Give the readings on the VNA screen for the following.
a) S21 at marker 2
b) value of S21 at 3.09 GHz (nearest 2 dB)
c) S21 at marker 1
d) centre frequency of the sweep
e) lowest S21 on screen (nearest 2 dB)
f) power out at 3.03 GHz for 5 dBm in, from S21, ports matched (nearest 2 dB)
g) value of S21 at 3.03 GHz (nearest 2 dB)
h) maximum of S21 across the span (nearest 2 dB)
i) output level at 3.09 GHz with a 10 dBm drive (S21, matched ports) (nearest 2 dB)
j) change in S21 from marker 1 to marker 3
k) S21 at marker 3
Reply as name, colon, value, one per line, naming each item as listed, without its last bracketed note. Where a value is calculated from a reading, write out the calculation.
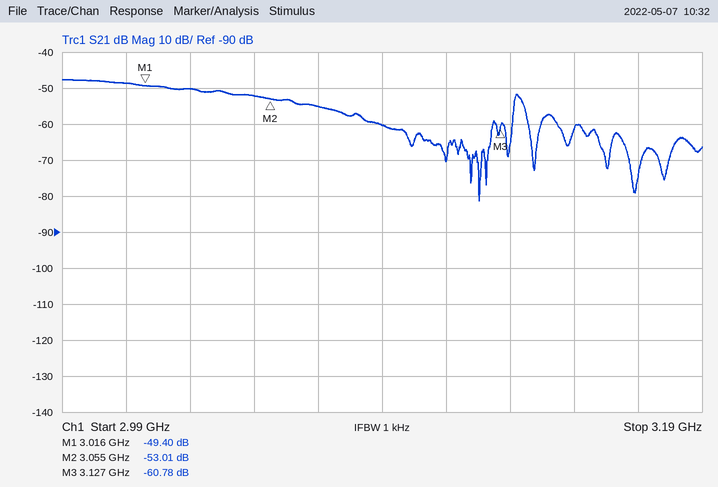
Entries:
S21 at marker 2: -53.01 dB
value of S21 at 3.09 GHz: -60 dB
S21 at marker 1: -49.40 dB
centre frequency of the sweep: 3.09 GHz
lowest S21 on screen: -82 dB
power out at 3.03 GHz for 5 dBm in, from S21, ports matched: 5 dBm + (-50 dB) = -46 dBm
value of S21 at 3.03 GHz: -50 dB
maximum of S21 across the span: -48 dB
output level at 3.09 GHz with a 10 dBm drive (S21, matched ports): 10 dBm + (-60 dB) = -50 dBm
change in S21 from marker 1 to marker 3: -60.78 − (-49.4) = -11.38 dB
S21 at marker 3: -60.78 dB
